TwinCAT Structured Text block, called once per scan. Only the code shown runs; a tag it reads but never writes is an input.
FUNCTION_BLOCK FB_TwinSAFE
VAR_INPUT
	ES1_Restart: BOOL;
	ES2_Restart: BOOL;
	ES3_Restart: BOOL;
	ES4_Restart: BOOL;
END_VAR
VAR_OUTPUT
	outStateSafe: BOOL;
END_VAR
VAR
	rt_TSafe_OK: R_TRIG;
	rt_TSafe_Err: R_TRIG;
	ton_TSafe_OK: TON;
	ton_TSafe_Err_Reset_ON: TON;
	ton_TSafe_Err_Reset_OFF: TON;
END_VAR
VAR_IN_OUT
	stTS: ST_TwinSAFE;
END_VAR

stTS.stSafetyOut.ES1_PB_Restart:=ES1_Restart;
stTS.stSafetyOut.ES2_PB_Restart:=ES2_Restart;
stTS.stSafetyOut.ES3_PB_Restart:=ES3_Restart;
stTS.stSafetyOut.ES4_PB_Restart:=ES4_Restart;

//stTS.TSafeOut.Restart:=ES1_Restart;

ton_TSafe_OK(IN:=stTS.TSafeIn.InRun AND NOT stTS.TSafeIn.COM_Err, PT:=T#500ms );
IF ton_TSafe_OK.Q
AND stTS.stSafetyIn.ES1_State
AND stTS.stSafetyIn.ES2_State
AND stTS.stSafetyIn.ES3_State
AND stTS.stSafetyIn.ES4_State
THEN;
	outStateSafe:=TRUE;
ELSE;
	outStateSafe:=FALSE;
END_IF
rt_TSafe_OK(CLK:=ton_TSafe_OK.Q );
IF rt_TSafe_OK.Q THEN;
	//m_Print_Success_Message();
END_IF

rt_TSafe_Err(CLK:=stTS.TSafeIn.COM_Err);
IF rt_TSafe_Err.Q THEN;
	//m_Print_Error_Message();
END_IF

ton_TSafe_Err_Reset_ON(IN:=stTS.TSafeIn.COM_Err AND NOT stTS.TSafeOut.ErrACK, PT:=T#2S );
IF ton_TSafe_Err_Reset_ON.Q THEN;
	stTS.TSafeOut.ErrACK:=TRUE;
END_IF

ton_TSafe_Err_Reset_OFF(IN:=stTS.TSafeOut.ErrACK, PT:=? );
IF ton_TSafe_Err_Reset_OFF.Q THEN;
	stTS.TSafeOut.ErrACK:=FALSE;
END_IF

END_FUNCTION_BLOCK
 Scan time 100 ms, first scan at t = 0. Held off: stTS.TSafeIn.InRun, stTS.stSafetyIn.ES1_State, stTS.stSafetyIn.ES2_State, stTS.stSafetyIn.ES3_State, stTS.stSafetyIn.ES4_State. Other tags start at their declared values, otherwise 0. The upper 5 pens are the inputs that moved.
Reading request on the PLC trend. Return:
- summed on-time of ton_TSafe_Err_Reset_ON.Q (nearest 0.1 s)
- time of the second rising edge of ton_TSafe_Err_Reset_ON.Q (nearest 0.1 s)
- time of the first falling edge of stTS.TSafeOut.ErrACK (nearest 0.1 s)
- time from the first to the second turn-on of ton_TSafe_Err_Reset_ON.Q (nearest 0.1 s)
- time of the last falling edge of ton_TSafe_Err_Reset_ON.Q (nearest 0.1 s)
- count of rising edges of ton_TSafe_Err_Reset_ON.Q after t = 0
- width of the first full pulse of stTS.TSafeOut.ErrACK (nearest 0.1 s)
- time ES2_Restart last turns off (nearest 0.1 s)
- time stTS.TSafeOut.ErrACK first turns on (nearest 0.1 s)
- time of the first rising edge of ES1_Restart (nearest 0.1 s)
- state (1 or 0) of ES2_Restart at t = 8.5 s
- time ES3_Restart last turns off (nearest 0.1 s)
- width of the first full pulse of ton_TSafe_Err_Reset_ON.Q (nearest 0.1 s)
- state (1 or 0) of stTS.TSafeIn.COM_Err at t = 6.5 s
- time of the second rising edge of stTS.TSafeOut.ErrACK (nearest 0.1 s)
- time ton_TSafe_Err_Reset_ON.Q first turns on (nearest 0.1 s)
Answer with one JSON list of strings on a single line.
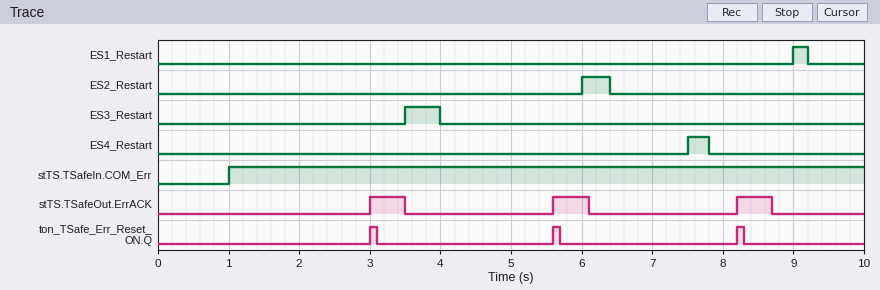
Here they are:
["0.3 s", "5.6 s", "3.5 s", "2.6 s", "8.3 s", "3", "0.5 s", "6.4 s", "3.0 s", "9.0 s", "0", "4.0 s", "0.1 s", "1", "5.6 s", "3.0 s"]
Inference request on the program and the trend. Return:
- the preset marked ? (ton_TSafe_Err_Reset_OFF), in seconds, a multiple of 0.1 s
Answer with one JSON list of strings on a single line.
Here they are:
["0.5 s"]
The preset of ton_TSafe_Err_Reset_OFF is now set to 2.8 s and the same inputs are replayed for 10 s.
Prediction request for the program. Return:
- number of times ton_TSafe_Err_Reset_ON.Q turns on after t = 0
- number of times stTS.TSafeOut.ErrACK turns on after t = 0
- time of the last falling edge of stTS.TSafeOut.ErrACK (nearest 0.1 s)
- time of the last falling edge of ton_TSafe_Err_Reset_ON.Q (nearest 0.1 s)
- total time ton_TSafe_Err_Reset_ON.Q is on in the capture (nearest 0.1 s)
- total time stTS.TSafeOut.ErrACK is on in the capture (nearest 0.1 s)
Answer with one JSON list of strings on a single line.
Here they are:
["2", "2", "5.8 s", "8.0 s", "0.2 s", "4.9 s"]
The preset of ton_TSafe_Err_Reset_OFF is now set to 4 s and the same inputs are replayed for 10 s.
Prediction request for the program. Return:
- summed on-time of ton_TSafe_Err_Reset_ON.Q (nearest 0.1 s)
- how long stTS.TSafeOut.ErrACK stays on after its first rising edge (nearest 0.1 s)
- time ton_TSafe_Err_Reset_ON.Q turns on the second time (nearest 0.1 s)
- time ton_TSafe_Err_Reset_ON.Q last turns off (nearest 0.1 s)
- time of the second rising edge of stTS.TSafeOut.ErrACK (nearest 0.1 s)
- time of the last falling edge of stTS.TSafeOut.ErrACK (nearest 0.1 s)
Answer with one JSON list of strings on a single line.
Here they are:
["0.2 s", "4.0 s", "9.1 s", "9.2 s", "9.1 s", "7.0 s"]
